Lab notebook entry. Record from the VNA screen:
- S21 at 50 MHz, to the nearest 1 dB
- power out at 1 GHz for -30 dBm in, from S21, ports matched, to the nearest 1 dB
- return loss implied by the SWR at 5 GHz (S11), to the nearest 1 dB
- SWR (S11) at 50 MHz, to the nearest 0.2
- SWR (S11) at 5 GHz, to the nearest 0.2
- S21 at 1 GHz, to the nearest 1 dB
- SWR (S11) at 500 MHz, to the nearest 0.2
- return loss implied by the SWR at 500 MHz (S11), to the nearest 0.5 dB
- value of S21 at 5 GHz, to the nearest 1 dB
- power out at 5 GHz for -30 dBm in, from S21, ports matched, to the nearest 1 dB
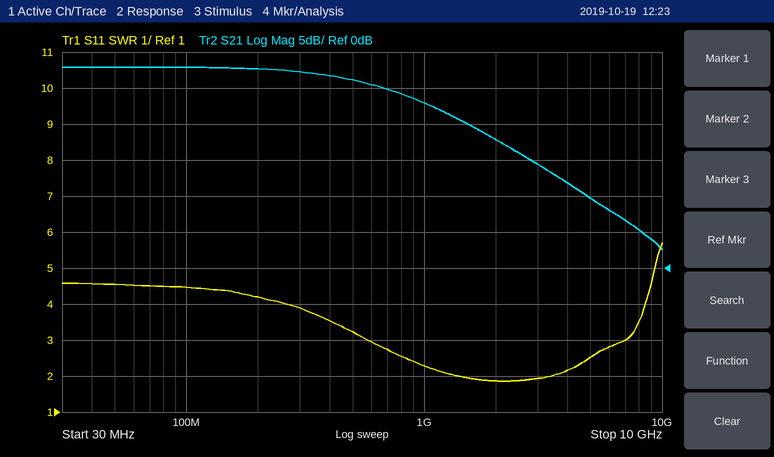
28 dB
-7 dBm
7 dB
4.6
2.6
23 dB
3.2
5.5 dB
10 dB
-20 dBm
